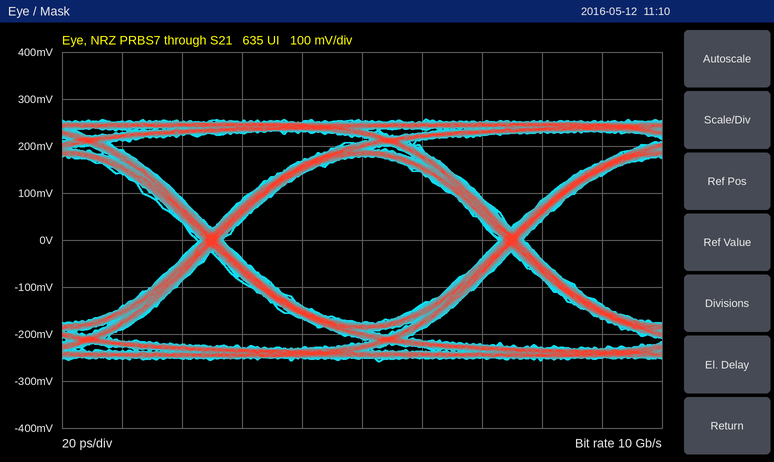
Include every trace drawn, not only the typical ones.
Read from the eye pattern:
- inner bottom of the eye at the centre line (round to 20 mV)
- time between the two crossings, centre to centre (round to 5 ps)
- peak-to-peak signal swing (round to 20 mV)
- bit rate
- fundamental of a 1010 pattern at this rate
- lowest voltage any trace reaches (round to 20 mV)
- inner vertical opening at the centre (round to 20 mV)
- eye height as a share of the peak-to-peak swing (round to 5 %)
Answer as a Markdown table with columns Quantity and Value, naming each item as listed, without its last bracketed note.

| Quantity | Value |
|---|---|
| inner bottom of the eye at the centre line | -180 mV |
| time between the two crossings, centre to centre | 100 ps |
| peak-to-peak signal swing | 520 mV |
| bit rate | 10 Gb/s |
| fundamental of a 1010 pattern at this rate | 5 GHz |
| lowest voltage any trace reaches | -260 mV |
| inner vertical opening at the centre | 360 mV |
| eye height as a share of the peak-to-peak swing | 70 % |
